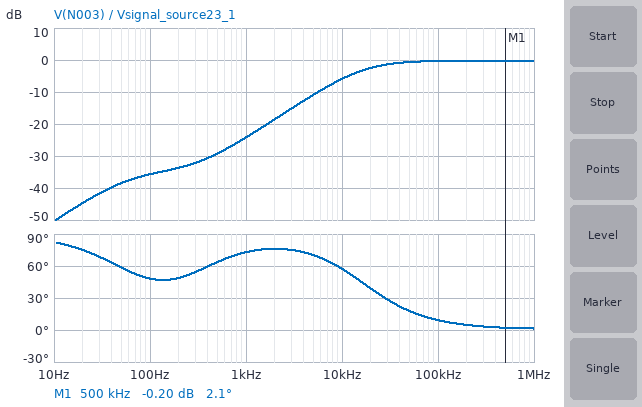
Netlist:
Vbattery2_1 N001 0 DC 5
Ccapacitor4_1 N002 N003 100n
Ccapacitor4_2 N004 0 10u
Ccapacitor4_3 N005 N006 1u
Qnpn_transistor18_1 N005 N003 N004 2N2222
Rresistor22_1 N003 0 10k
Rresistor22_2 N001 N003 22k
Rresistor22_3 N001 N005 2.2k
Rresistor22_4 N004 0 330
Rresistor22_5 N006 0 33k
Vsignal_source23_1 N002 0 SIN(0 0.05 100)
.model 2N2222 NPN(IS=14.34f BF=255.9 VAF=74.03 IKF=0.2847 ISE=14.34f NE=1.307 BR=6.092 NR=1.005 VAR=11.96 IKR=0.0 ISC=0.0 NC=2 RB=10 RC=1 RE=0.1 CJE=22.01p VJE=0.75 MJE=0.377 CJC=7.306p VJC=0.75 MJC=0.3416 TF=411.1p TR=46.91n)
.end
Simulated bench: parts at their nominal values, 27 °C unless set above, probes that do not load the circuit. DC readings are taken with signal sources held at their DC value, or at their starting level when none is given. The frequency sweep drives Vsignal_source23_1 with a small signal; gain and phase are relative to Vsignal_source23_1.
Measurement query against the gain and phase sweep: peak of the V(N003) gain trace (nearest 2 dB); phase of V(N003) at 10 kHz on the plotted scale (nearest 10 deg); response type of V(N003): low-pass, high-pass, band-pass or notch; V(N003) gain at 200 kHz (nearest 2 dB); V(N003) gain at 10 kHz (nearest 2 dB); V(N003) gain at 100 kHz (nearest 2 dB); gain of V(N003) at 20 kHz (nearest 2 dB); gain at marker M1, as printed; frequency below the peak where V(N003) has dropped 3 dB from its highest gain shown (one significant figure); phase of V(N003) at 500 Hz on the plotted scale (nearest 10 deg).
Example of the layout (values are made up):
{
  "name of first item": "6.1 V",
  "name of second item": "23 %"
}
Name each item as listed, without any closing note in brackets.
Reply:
{
  "peak of the V(N003) gain trace": "0 dB",
  "phase of V(N003) at 10 kHz on the plotted scale": "60 deg",
  "response type of V(N003): low-pass, high-pass, band-pass or notch": "high-pass",
  "V(N003) gain at 200 kHz": "0 dB",
  "V(N003) gain at 10 kHz": "-6 dB",
  "V(N003) gain at 100 kHz": "0 dB",
  "gain of V(N003) at 20 kHz": "-2 dB",
  "gain at marker M1, as printed": "-0.20 dB",
  "frequency below the peak where V(N003) has dropped 3 dB from its highest gain shown": "20 kHz",
  "phase of V(N003) at 500 Hz on the plotted scale": "60 deg"
}
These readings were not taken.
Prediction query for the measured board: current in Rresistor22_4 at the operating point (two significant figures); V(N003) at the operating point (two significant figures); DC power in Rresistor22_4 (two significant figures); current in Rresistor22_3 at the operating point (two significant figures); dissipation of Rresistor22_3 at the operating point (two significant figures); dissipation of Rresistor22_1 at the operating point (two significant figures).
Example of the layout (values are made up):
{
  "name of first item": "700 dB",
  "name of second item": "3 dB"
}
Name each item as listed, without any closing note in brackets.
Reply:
{
  "current in Rresistor22_4 at the operating point": "2.0 mA",
  "V(N003) at the operating point": "1.3 V",
  "DC power in Rresistor22_4": "1.3 mW",
  "current in Rresistor22_3 at the operating point": "1.9 mA",
  "dissipation of Rresistor22_3 at the operating point": "8.3 mW",
  "dissipation of Rresistor22_1 at the operating point": "170 µW"
}
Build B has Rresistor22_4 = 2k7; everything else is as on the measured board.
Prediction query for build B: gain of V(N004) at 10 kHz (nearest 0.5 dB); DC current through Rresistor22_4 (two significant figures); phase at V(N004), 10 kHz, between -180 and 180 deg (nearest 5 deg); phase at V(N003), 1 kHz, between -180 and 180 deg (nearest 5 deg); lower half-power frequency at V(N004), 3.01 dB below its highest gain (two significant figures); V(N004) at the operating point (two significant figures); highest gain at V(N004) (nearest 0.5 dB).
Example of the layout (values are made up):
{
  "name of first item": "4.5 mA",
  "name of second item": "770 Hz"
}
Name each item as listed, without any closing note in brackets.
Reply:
{
  "gain of V(N004) at 10 kHz": "-33.5 dB",
  "DC current through Rresistor22_4": "340 µA",
  "phase at V(N004), 10 kHz, between -180 and 180 deg": "-85 deg",
  "phase at V(N003), 1 kHz, between -180 and 180 deg": "20 deg",
  "lower half-power frequency at V(N004), 3.01 dB below its highest gain": "76 Hz",
  "V(N004) at the operating point": "930 mV",
  "highest gain at V(N004)": "-9.0 dB"
}
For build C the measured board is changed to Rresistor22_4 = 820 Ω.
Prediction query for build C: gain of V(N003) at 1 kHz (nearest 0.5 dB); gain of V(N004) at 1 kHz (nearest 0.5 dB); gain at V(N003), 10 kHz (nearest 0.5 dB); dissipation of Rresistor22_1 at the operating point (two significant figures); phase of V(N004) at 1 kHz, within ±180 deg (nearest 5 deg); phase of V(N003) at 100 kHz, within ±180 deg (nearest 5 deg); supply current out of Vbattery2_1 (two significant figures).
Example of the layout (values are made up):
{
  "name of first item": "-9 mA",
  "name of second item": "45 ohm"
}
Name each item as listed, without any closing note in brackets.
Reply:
{
  "gain of V(N003) at 1 kHz": "-2.0 dB",
  "gain of V(N004) at 1 kHz": "-8.0 dB",
  "gain at V(N003), 10 kHz": "0 dB",
  "dissipation of Rresistor22_1 at the operating point": "230 µW",
  "phase of V(N004) at 1 kHz, within ±180 deg": "-35 deg",
  "phase of V(N003) at 100 kHz, within ±180 deg": "0 deg",
  "supply current out of Vbattery2_1": "1.2 mA"
}
